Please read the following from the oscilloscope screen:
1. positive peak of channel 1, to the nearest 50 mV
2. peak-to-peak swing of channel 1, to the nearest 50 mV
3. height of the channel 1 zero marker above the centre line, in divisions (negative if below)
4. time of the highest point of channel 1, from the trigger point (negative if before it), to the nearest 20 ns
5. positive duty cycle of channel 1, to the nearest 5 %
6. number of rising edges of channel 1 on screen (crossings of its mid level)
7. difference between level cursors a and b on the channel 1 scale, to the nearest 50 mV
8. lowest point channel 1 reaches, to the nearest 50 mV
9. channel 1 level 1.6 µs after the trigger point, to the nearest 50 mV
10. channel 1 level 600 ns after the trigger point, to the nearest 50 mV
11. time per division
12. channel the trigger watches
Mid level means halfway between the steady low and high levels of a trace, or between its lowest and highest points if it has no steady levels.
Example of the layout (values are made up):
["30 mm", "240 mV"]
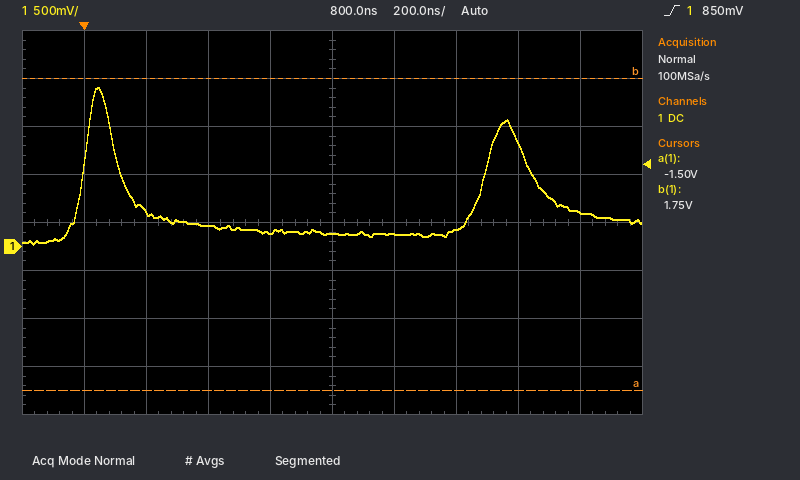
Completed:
["1.65 V", "1.65 V", "-0.5 div", "+40 ns", "10 %", "2", "3.25 V", "0 mV", "350 mV", "150 mV", "200 ns", "channel 1"]
